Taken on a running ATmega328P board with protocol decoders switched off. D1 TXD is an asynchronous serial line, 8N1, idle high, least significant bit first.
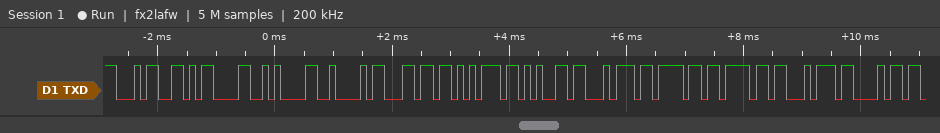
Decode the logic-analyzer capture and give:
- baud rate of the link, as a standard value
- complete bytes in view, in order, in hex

9600 baud
0x34 0x0D 0x0A 0x42 0x6C 0x75 0x65 0x74 0x6F 0x6F 0x74 0x68
